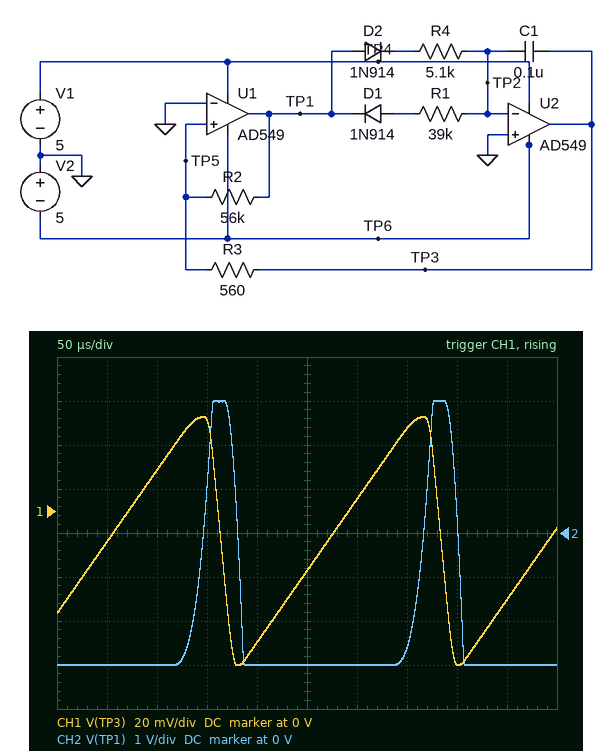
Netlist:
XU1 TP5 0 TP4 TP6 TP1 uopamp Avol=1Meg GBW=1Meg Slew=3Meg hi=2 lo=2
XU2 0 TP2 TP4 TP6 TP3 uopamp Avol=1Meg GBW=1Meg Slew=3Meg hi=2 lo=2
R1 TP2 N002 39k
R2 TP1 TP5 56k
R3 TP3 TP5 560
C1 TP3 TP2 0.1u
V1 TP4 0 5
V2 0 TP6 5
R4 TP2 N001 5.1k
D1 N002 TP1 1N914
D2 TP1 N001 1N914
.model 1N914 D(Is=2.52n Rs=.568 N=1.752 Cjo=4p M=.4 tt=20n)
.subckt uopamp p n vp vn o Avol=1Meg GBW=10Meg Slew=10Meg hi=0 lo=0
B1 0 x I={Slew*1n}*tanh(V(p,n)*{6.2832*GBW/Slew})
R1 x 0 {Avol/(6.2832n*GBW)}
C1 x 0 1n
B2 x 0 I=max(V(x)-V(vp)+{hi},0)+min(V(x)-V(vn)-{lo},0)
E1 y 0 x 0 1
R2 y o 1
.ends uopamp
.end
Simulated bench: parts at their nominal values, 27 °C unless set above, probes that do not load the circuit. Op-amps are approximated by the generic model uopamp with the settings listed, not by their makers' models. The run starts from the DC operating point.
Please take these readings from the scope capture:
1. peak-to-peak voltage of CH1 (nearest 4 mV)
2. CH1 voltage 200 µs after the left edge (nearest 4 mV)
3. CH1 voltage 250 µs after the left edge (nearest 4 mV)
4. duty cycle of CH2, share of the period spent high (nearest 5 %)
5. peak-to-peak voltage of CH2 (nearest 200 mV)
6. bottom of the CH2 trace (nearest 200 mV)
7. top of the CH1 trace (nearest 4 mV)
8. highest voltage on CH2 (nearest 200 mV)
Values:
112 mV
-60 mV
-28 mV
15 %
6.0 V
-3.0 V
44 mV
3.0 V
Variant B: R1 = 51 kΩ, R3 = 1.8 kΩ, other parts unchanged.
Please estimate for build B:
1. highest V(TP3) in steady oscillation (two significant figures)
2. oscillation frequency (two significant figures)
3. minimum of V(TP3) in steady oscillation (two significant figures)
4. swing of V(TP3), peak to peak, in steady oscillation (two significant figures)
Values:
100 mV
1.9 kHz
-130 mV
230 mV
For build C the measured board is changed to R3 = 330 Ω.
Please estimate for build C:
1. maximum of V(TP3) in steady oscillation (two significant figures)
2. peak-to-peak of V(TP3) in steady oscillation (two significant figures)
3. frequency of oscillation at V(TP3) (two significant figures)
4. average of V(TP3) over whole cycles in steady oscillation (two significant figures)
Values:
32 mV
91 mV
5.3 kHz
-12 mV
